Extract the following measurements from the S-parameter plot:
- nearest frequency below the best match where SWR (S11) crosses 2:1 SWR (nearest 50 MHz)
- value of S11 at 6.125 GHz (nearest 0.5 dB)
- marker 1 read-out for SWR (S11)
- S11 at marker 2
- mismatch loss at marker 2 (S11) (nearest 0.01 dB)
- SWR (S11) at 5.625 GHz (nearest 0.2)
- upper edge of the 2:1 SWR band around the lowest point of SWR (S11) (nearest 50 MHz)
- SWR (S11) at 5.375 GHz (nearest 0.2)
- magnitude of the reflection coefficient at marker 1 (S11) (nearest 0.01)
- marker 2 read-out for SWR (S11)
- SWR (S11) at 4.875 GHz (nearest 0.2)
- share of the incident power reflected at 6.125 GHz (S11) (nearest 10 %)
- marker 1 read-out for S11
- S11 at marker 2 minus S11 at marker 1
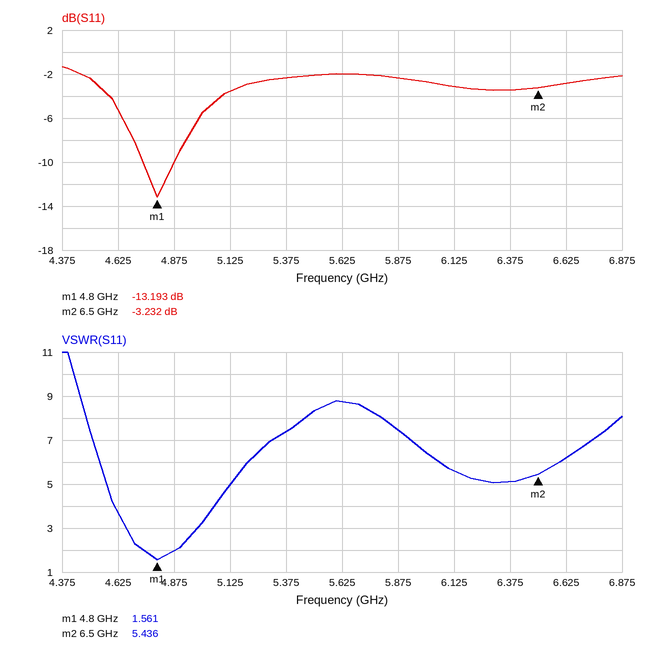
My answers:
4.75 GHz
-3.0 dB
1.561
-3.232 dB
2.80 dB
8.8
4.90 GHz
7.4
0.22
5.436
2.0
50 %
-13.193 dB
9.961 dB
